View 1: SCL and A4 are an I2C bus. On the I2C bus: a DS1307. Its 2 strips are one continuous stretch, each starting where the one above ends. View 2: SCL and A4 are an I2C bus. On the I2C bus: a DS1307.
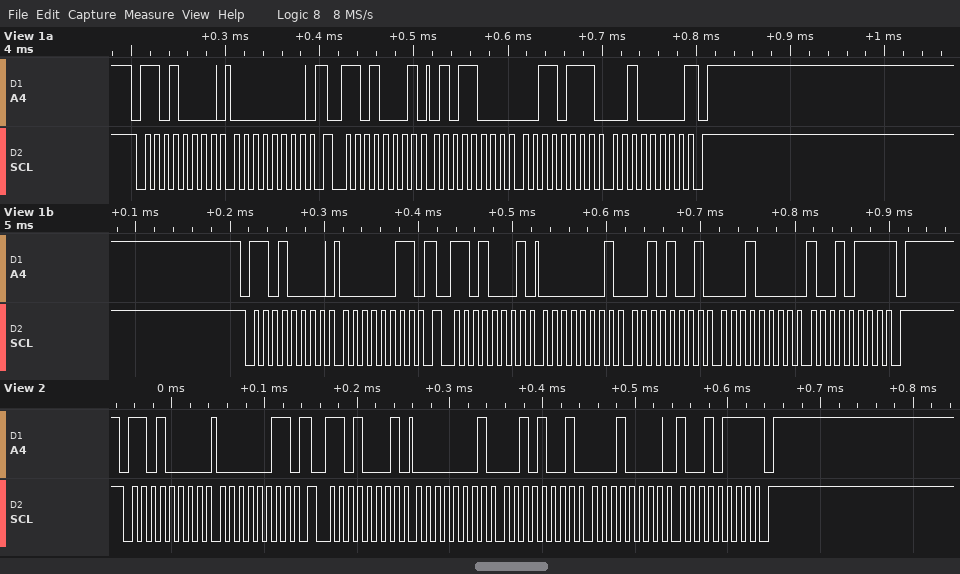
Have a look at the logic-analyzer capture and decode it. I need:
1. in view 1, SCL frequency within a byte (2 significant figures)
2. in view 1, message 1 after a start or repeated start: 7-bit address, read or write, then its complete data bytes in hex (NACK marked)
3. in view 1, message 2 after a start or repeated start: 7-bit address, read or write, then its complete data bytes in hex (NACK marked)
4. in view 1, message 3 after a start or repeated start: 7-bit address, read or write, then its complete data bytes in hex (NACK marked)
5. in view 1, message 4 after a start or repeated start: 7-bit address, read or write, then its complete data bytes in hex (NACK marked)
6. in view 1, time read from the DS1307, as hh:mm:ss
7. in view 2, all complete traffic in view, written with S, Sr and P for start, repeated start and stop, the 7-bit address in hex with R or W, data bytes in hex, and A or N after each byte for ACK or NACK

100 kHz
0x68 write: 00
0x68 read: 58 37 20 NACK
0x68 write: 03
0x68 read: 01 29 10 97 NACK
20:37:58
S 68W A 03 A Sr 68R A 01 A 29 A 10 A 97 N P
